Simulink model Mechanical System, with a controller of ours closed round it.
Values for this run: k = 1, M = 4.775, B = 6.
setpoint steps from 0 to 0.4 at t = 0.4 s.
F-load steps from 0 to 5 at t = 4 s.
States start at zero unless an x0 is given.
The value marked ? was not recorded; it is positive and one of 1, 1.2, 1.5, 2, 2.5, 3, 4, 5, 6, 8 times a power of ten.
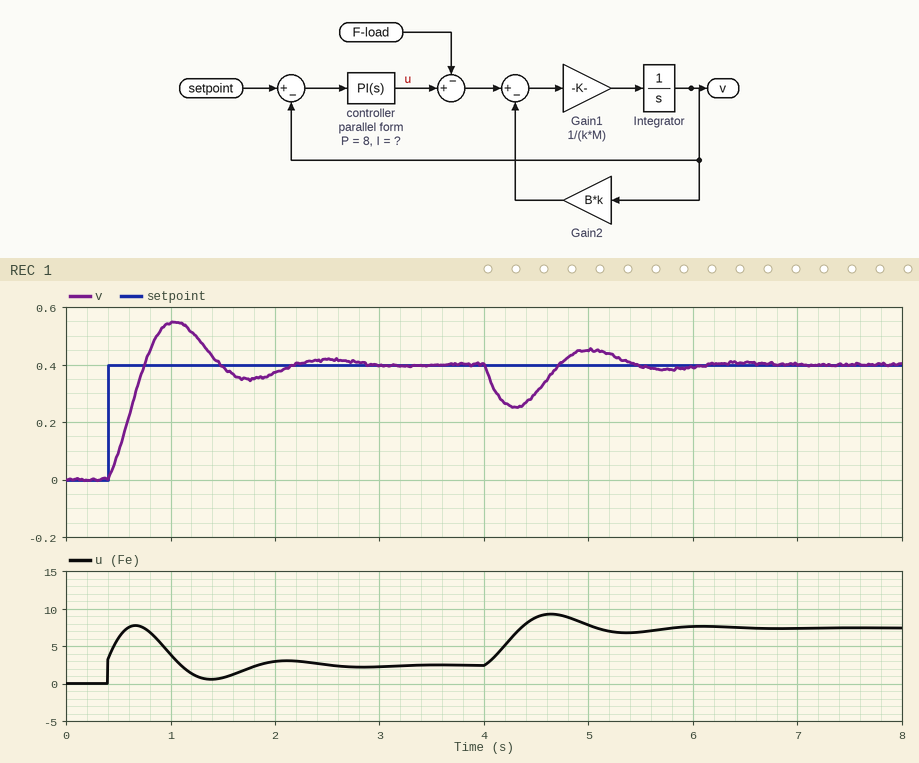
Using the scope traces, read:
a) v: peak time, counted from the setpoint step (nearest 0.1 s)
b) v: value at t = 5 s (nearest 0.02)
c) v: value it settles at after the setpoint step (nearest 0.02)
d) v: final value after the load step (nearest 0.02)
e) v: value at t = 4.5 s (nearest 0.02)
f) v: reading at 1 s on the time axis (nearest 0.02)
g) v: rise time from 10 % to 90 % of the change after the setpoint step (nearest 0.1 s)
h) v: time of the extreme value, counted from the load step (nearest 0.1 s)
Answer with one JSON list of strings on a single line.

["0.6 s", "0.46", "0.40", "0.40", "0.30", "0.54", "0.3 s", "0.3 s"]
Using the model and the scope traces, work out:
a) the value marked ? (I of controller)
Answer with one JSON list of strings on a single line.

["100"]
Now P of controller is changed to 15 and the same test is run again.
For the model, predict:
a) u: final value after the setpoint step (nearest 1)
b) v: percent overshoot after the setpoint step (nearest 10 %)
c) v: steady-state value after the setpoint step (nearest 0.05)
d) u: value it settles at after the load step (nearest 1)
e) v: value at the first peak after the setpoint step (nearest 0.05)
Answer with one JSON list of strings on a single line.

["2", "20 %", "0.40", "7", "0.50"]
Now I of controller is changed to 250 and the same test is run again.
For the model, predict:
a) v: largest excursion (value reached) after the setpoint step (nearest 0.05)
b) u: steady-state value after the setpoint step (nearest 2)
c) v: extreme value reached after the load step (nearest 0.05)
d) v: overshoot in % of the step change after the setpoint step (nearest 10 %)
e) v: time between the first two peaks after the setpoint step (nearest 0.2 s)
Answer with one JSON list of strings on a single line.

["0.60", "2", "0.30", "50 %", "0.8 s"]
